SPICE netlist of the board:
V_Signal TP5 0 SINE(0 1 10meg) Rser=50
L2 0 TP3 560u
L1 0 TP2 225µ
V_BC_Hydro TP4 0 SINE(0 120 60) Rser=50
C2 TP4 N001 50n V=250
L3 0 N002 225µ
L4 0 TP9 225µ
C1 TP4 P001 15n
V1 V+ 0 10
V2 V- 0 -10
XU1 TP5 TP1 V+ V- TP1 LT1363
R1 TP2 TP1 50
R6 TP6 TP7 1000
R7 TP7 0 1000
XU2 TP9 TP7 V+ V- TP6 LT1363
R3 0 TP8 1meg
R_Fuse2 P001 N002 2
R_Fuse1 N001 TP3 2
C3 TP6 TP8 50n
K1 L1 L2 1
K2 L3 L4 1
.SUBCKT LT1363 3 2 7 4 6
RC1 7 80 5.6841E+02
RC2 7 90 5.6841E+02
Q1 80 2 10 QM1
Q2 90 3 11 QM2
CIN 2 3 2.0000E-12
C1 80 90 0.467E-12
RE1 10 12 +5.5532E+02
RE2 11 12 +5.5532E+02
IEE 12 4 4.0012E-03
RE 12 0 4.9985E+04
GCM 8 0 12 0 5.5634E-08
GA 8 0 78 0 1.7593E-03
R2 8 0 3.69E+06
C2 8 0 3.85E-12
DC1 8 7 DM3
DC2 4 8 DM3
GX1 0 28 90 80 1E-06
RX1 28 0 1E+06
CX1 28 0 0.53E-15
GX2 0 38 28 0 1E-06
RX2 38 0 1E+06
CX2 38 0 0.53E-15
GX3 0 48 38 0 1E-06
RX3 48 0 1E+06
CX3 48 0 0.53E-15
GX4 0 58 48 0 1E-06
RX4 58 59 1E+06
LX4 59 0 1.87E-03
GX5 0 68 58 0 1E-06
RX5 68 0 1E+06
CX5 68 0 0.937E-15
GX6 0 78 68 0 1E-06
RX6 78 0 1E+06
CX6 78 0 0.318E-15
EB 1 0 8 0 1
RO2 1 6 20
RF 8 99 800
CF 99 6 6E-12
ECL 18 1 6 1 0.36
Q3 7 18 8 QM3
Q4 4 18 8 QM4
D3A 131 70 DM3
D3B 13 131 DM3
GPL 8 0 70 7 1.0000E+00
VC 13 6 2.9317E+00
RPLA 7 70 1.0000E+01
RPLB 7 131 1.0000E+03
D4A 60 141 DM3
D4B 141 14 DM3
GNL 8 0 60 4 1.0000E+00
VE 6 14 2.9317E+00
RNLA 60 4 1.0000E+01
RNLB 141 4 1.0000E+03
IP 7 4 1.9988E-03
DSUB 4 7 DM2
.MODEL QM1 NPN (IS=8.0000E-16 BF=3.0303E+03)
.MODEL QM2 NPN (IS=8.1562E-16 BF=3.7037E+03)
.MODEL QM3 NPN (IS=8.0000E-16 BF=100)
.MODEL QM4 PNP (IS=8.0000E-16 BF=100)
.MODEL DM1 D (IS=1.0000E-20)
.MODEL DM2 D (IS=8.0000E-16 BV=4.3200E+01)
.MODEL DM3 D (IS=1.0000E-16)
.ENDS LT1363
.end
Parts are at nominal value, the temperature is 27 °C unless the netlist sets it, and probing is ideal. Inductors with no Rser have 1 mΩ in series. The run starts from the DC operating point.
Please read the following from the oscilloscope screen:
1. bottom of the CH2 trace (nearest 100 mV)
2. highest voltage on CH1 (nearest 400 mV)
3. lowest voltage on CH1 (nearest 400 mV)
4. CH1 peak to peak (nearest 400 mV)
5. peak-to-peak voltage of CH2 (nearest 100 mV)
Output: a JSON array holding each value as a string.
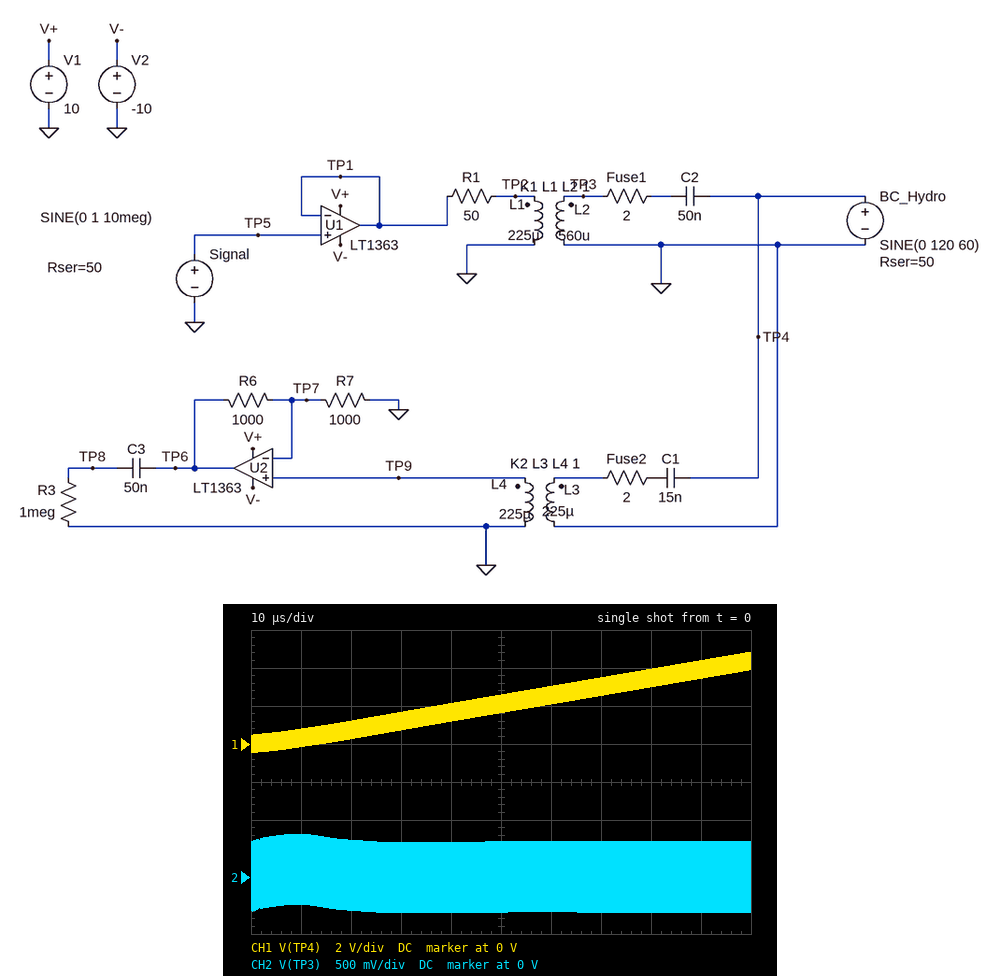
["-500 mV", "4.8 V", "-400 mV", "5.2 V", "1.0 V"]
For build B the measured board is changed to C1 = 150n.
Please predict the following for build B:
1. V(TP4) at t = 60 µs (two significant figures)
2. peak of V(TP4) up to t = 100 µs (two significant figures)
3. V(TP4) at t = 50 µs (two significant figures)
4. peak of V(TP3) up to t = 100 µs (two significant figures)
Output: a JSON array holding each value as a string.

["2.2 V", "4.5 V", "1.7 V", "520 mV"]
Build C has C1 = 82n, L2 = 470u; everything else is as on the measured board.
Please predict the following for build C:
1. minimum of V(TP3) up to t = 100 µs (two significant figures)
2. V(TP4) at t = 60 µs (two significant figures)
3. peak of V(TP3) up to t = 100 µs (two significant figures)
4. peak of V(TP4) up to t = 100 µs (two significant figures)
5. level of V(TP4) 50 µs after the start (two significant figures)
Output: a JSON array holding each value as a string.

["-480 mV", "2.3 V", "530 mV", "4.7 V", "1.9 V"]
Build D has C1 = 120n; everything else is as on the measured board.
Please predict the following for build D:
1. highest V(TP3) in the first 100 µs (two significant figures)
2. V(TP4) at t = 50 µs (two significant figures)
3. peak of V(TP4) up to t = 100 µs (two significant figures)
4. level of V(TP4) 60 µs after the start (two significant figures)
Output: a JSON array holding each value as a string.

["520 mV", "1.8 V", "4.6 V", "2.2 V"]
